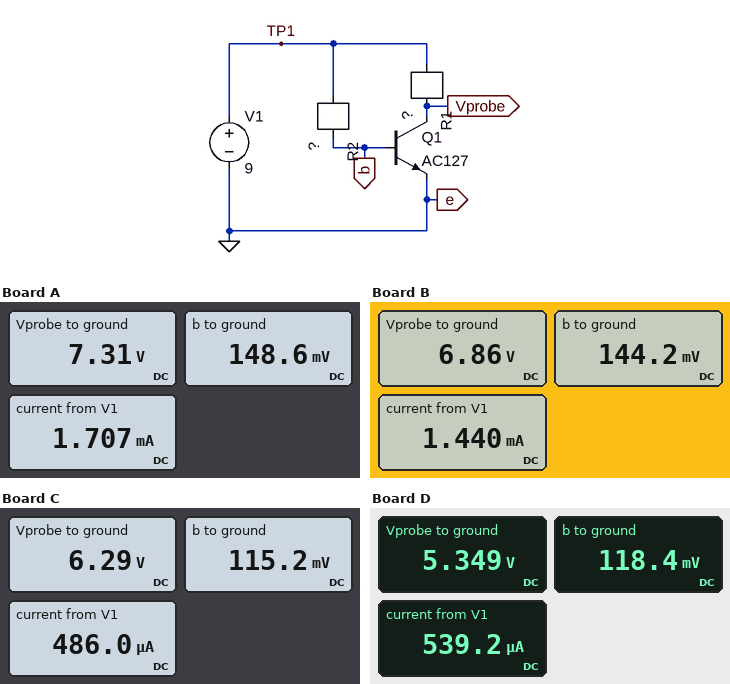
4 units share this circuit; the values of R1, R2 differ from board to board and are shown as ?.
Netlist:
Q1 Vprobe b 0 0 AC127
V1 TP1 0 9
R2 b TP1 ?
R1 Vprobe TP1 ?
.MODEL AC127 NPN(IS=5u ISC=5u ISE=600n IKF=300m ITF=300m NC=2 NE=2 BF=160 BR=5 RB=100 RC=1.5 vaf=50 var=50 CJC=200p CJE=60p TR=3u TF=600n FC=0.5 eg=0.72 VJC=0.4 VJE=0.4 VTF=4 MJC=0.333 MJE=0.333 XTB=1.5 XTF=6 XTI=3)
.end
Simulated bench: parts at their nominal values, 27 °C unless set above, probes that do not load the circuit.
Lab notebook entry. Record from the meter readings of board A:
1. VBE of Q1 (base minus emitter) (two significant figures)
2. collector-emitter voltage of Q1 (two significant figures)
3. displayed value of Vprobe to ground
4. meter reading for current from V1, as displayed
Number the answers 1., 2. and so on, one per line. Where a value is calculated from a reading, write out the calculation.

1. 148.6 mV = 150 mV
2. 7.31 V = 7.3 V
3. 7.31 V
4. 1.707 mA
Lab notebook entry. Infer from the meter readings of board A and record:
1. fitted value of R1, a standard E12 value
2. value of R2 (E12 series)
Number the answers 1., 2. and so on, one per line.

1. 1 kΩ
2. 680 kΩ
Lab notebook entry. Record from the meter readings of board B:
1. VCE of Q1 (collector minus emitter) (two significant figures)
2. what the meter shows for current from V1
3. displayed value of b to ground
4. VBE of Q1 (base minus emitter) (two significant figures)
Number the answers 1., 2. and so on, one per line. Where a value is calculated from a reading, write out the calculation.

1. 6.86 V = 6.9 V
2. 1.440 mA
3. 144.2 mV
4. 144.2 mV = 140 mV
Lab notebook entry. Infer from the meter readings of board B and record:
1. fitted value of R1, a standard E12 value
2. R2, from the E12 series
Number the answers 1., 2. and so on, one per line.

1. 1.5 kΩ
2. 820 kΩ
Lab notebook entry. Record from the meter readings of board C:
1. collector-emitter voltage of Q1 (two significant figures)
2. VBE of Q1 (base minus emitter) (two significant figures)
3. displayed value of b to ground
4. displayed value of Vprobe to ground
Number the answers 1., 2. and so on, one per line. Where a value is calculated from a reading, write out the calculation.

1. 6.29 V = 6.3 V
2. 115.2 mV = 120 mV
3. 115.2 mV
4. 6.29 V
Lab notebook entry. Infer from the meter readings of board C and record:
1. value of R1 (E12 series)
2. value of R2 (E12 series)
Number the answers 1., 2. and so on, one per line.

1. 5.6 kΩ
2. 5.6 MΩ
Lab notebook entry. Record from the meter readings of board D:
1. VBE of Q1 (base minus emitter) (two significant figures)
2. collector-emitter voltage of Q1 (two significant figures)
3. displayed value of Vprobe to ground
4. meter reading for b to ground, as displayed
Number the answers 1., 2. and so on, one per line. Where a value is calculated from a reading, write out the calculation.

1. 118.4 mV = 120 mV
2. 5.349 V = 5.3 V
3. 5.349 V
4. 118.4 mV
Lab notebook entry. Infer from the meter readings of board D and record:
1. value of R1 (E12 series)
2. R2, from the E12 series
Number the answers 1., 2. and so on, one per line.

1. 6.8 kΩ
2. 3.9 MΩ
